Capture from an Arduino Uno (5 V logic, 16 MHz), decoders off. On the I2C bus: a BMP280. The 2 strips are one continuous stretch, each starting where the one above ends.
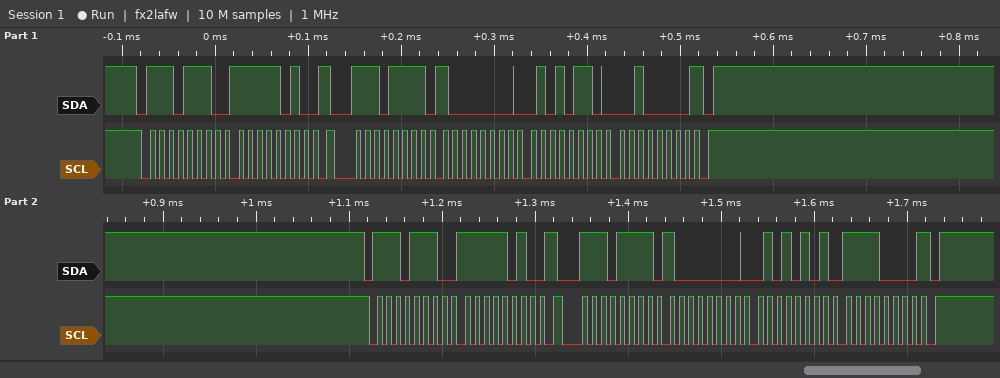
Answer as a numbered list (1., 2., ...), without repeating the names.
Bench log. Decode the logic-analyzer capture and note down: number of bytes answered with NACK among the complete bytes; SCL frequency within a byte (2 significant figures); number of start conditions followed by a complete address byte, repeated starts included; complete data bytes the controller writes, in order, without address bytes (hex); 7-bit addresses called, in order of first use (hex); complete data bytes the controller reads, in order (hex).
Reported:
1. 2
2. 100 kHz
3. 4
4. FA FA
5. 0x77
6. 80 56 20 80 55 F0
